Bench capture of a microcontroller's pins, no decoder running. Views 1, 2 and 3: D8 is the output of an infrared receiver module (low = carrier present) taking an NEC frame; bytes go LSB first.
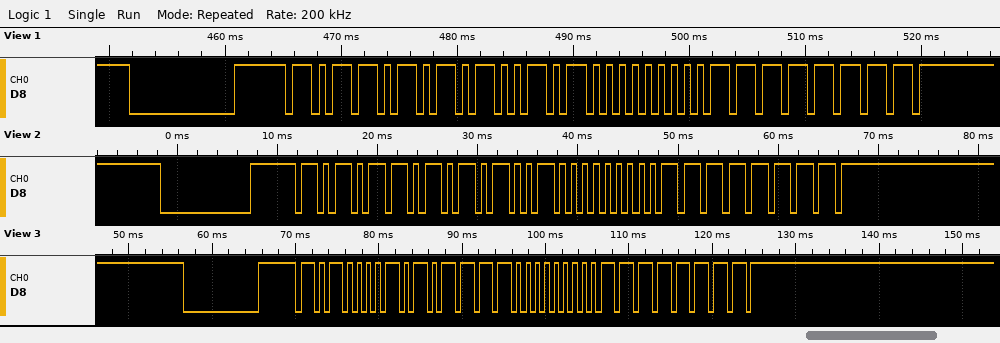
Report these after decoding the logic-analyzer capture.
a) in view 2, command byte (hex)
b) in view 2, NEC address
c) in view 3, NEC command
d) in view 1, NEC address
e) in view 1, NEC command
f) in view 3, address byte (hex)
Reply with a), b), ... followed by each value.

a) 0x00
b) 0xB5
c) 0x00
d) 0xAD
e) 0x00
f) 0x85
